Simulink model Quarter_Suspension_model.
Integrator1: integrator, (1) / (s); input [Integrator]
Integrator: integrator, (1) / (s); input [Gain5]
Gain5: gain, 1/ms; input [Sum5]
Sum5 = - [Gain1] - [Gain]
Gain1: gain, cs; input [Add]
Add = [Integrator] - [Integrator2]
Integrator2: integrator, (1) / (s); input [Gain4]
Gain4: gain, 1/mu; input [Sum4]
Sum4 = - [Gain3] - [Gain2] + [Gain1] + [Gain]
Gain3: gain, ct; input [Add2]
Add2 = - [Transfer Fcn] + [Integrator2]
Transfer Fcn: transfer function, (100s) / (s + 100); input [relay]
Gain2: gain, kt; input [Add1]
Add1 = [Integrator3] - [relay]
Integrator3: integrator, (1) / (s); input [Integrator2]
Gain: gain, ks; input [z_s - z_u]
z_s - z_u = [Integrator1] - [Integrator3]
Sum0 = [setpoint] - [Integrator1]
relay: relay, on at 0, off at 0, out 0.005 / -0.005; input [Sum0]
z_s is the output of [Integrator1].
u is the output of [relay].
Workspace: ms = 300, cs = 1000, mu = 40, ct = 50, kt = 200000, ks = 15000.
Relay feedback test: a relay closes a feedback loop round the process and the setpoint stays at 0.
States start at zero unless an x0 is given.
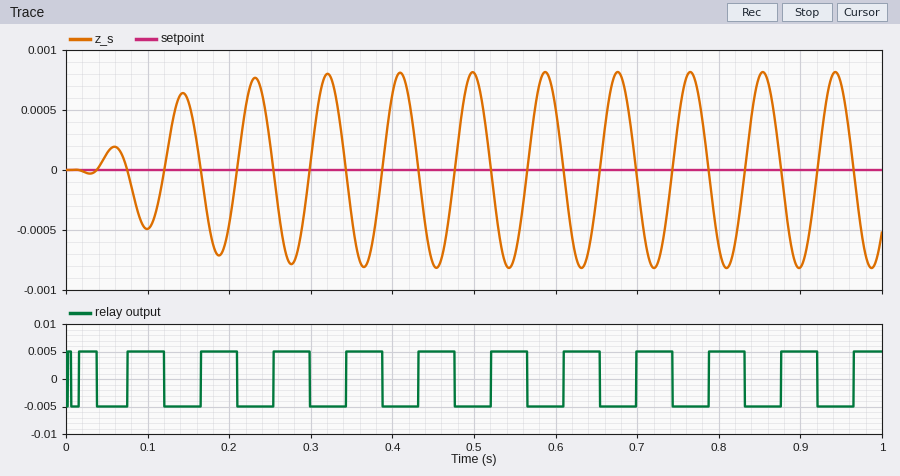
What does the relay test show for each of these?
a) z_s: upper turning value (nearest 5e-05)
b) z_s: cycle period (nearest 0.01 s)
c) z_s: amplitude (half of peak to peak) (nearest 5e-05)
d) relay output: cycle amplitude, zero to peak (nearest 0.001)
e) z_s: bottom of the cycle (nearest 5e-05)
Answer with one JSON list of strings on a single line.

["0.00080", "0.09 s", "0.00080", "0.005", "-0.00080"]
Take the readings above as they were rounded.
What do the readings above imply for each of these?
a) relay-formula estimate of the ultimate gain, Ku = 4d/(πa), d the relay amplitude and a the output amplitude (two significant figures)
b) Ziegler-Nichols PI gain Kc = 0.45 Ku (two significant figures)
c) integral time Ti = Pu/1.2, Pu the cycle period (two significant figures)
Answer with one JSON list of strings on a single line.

["8.0", "3.6", "0.075 s"]
